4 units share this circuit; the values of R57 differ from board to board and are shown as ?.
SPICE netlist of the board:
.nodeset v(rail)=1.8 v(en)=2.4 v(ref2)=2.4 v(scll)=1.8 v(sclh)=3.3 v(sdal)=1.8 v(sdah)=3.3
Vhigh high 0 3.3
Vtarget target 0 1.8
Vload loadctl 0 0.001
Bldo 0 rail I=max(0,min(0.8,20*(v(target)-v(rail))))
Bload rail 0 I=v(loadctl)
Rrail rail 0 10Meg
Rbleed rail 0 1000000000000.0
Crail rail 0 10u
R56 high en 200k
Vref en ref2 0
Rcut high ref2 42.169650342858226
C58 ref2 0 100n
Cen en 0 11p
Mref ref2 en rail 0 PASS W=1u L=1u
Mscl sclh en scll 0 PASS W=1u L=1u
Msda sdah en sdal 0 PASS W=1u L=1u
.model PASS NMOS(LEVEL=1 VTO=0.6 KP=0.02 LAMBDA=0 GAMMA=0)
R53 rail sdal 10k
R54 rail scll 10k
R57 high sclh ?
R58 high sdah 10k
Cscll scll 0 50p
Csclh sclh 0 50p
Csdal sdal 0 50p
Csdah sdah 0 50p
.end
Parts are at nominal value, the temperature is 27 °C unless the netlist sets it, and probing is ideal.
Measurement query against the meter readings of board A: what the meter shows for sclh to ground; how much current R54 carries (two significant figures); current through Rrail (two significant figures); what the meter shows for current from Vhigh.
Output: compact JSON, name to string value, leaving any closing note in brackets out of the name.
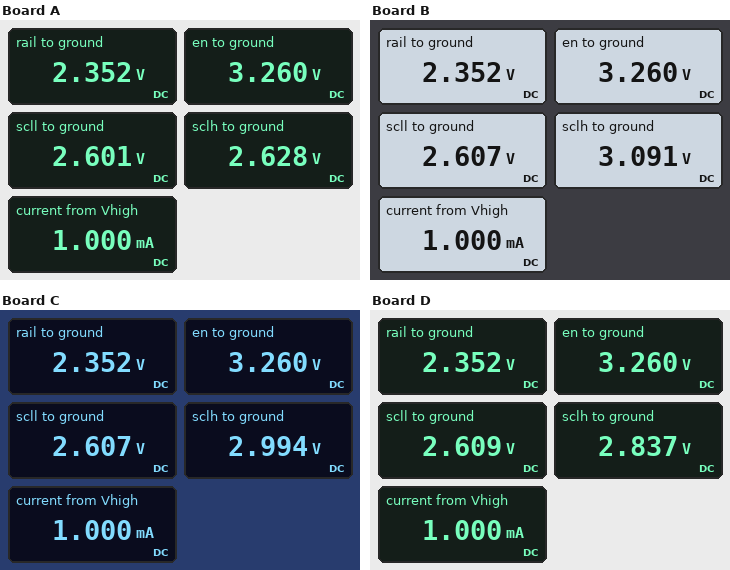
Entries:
{"what the meter shows for sclh to ground": "2.628 V", "how much current R54 carries": "25 µA", "current through Rrail": "240 nA", "what the meter shows for current from Vhigh": "1.000 mA"}
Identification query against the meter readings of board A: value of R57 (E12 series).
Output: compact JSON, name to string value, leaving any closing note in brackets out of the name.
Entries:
{"value of R57": "27 kΩ"}
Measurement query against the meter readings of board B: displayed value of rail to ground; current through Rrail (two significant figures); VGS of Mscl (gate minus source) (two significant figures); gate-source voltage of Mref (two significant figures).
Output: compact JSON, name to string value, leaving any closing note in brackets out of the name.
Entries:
{"displayed value of rail to ground": "2.352 V", "current through Rrail": "240 nA", "VGS of Mscl (gate minus source)": "650 mV", "gate-source voltage of Mref": "910 mV"}
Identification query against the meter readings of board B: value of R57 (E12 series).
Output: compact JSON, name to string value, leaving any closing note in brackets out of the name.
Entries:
{"value of R57": "8.2 kΩ"}
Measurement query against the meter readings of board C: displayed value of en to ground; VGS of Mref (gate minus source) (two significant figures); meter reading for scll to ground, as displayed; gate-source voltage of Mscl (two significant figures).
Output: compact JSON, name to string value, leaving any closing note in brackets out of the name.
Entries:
{"displayed value of en to ground": "3.260 V", "VGS of Mref (gate minus source)": "910 mV", "meter reading for scll to ground, as displayed": "2.607 V", "gate-source voltage of Mscl": "650 mV"}
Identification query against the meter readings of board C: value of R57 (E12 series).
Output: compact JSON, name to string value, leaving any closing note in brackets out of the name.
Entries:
{"value of R57": "12 kΩ"}
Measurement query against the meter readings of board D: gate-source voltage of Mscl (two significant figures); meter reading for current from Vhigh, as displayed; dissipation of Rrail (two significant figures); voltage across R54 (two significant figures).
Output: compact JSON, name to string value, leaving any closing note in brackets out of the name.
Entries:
{"gate-source voltage of Mscl": "650 mV", "meter reading for current from Vhigh, as displayed": "1.000 mA", "dissipation of Rrail": "550 nW", "voltage across R54": "260 mV"}
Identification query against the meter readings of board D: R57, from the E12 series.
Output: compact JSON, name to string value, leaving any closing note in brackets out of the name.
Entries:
{"R57, from the E12 series": "18 kΩ"}
